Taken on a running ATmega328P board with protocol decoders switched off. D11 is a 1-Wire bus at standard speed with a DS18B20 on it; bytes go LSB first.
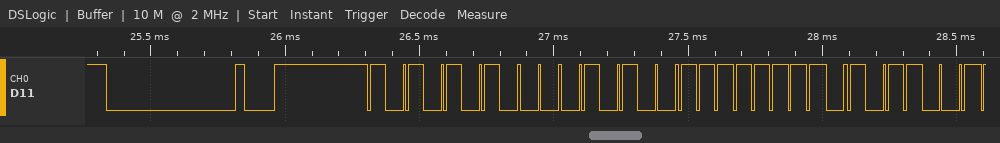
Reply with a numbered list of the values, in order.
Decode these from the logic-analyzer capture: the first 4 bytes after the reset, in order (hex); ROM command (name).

1. 55 28 FF 9A
2. Match ROM
